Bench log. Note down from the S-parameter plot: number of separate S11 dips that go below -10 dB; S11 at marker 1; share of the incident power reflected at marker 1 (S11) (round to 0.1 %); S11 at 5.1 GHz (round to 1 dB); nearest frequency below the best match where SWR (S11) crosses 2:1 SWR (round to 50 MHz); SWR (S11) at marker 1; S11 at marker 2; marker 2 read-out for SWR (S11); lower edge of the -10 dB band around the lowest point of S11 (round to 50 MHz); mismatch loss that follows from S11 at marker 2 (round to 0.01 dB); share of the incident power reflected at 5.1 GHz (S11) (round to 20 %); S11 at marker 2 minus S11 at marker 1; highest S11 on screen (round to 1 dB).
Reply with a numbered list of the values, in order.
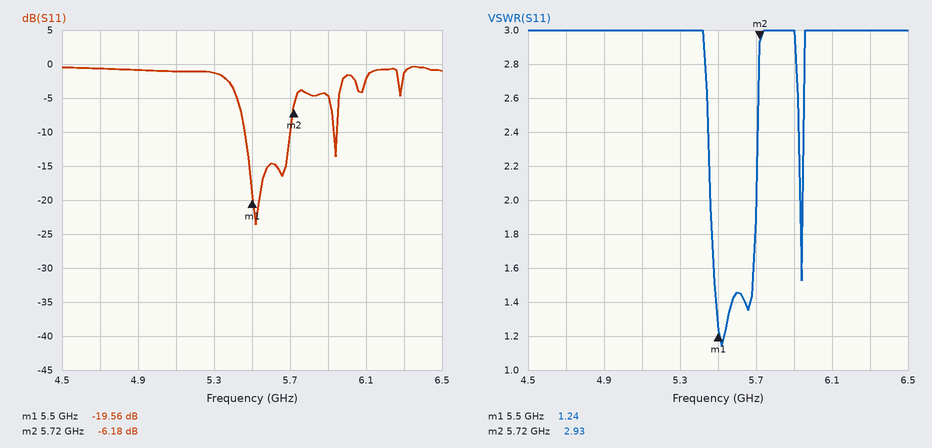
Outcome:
1. 2
2. -19.56 dB
3. 1.1 %
4. -1 dB
5. 5.45 GHz
6. 1.24
7. -6.18 dB
8. 2.93
9. 5.45 GHz
10. 1.20 dB
11. 80 %
12. 13.38 dB
13. 0 dB
